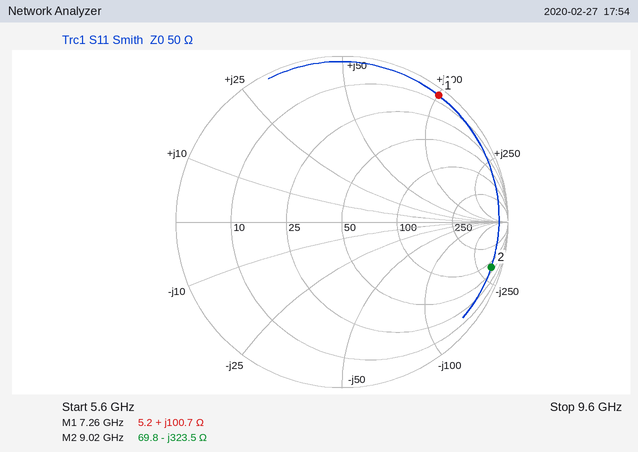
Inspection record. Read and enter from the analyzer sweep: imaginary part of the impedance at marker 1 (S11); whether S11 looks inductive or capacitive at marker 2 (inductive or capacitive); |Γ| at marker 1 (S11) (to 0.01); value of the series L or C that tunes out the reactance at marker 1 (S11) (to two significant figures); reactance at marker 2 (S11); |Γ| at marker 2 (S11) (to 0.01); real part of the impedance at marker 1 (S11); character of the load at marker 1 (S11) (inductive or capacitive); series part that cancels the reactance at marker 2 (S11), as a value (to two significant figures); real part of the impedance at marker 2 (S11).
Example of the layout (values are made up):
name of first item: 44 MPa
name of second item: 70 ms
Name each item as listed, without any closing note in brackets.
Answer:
imaginary part of the impedance at marker 1: +100.7 Ω
whether S11 looks inductive or capacitive at marker 2: capacitive
|Γ| at marker 1 (S11): 0.96
value of the series L or C that tunes out the reactance at marker 1 (S11): 220 fF
reactance at marker 2: -323.5 Ω
|Γ| at marker 2 (S11): 0.94
real part of the impedance at marker 1: 5.2 Ω
character of the load at marker 1 (S11): inductive
series part that cancels the reactance at marker 2 (S11), as a value: 5.7 nH
real part of the impedance at marker 2: 69.8 Ω
